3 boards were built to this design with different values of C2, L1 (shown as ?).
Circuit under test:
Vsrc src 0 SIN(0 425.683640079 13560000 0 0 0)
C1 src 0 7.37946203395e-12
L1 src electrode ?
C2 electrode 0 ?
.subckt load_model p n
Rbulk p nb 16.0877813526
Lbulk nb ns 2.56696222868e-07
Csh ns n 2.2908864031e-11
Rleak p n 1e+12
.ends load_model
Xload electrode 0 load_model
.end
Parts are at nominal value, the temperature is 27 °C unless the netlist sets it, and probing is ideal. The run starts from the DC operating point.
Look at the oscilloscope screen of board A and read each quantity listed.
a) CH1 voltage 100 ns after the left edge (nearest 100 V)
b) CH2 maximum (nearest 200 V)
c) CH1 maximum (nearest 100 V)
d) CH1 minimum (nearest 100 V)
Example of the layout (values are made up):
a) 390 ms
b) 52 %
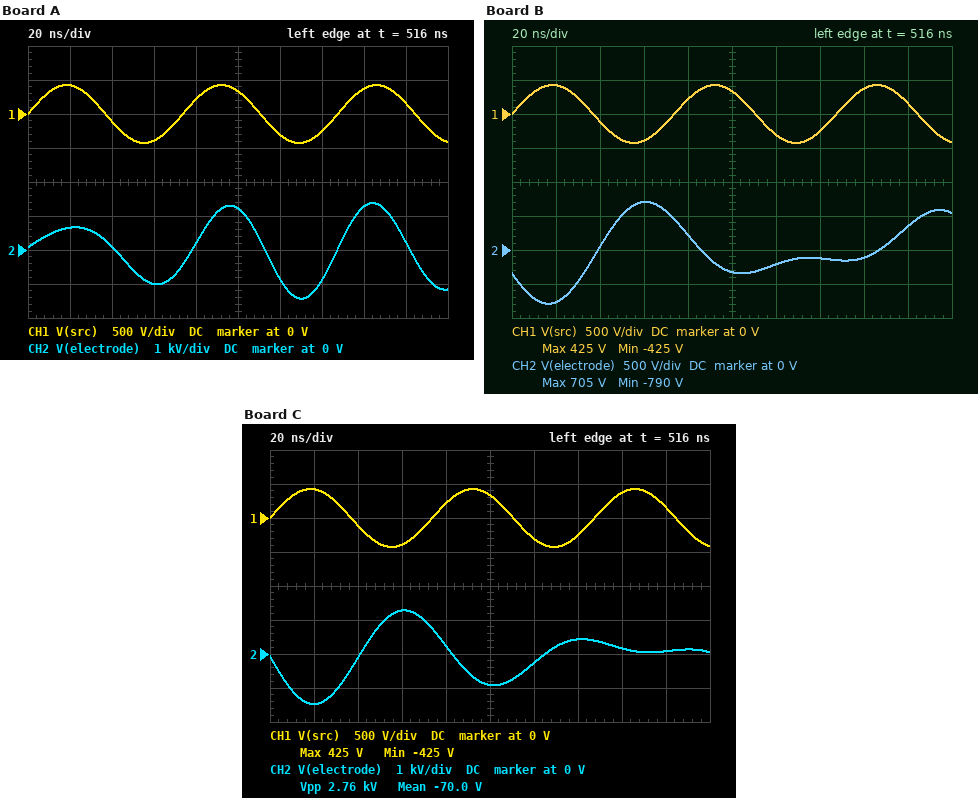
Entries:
a) 300 V
b) 1.4 kV
c) 400 V
d) -400 V
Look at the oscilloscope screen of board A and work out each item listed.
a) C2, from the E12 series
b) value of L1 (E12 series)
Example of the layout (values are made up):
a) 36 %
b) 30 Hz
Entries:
a) 22 pF
b) 1.8 µH
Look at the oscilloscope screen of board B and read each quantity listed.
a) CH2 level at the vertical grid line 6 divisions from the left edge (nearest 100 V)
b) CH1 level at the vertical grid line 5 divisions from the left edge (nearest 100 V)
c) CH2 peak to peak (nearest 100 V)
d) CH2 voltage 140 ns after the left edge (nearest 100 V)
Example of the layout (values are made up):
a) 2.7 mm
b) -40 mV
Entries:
a) -200 V
b) 300 V
c) 1.5 kV
d) -100 V
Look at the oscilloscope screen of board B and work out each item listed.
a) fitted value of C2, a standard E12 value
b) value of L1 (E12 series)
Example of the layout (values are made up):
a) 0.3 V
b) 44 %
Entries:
a) 120 pF
b) 2.2 µH
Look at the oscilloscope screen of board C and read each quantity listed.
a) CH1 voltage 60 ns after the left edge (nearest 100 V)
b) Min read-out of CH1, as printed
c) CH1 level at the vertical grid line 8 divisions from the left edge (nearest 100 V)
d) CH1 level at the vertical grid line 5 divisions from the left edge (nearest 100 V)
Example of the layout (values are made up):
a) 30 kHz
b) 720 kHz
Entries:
a) -400 V
b) -425 V
c) 400 V
d) 300 V
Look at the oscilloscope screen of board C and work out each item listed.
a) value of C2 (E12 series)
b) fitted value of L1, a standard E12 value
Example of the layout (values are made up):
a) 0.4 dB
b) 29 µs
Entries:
a) 100 pF
b) 1.8 µH
